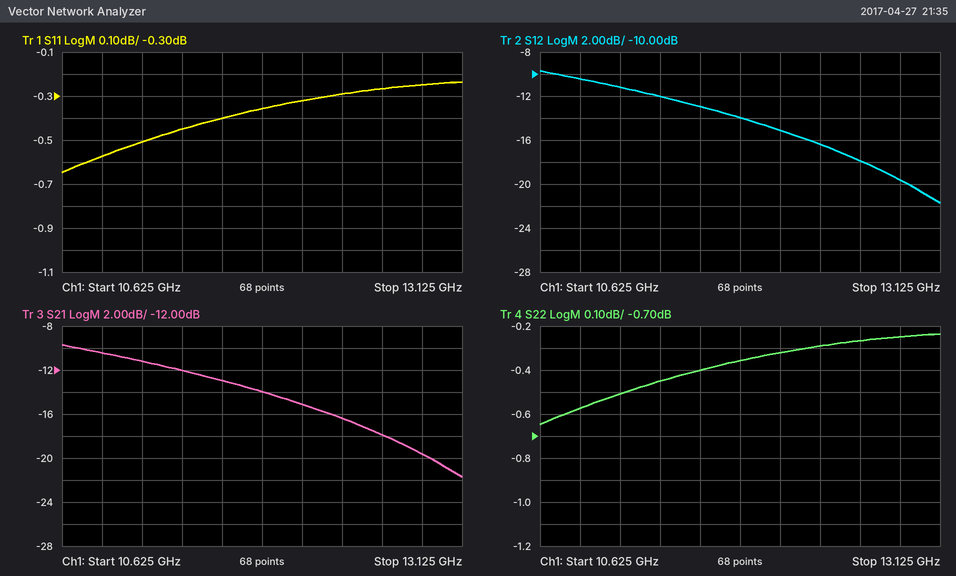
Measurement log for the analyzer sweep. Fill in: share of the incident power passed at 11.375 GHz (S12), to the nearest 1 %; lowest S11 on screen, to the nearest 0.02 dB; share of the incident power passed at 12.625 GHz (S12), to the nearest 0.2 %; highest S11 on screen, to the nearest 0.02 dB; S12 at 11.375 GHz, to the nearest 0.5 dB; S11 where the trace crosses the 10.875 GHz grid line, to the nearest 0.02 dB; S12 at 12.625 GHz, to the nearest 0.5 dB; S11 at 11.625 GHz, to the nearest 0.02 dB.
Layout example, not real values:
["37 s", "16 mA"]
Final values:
["6 %", "-0.64 dB", "1.6 %", "-0.24 dB", "-12.0 dB", "-0.58 dB", "-18.0 dB", "-0.40 dB"]
